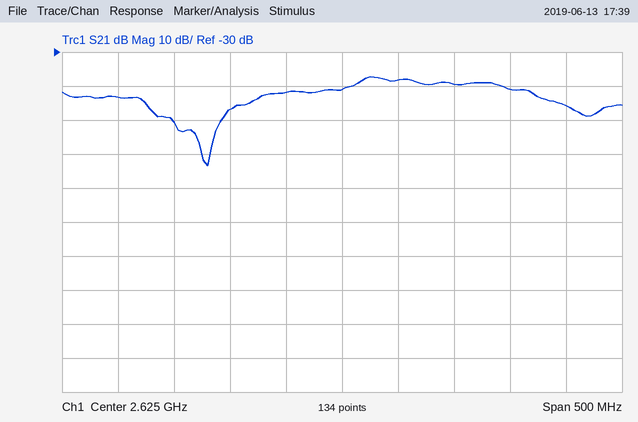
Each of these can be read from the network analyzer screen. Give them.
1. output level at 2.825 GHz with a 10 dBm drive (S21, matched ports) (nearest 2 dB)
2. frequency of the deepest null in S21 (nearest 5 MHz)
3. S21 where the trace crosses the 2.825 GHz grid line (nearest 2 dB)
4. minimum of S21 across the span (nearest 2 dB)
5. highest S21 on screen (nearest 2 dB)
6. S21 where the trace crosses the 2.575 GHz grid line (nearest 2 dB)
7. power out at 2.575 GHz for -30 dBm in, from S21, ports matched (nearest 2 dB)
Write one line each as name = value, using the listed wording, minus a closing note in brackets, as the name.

output level at 2.825 GHz with a 10 dBm drive (S21, matched ports) = -36 dBm
frequency of the deepest null in S21 = 2.505 GHz
S21 where the trace crosses the 2.825 GHz grid line = -46 dB
minimum of S21 across the span = -64 dB
highest S21 on screen = -38 dB
S21 where the trace crosses the 2.575 GHz grid line = -42 dB
power out at 2.575 GHz for -30 dBm in, from S21, ports matched = -72 dBm
